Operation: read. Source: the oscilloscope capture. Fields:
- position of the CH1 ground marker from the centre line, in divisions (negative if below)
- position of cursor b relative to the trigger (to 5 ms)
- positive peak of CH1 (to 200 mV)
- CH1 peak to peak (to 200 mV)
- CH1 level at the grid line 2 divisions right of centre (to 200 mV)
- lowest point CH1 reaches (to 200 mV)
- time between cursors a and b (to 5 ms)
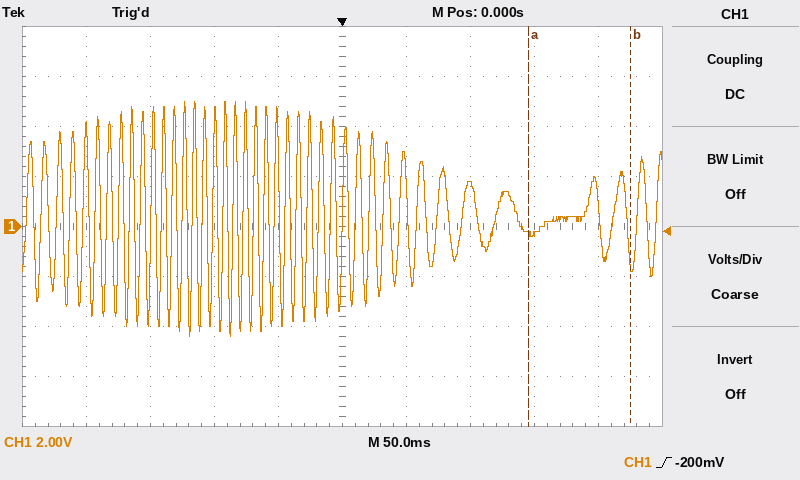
0.0 div
+225 ms
5.0 V
9.4 V
1.6 V
-4.4 V
80 ms
